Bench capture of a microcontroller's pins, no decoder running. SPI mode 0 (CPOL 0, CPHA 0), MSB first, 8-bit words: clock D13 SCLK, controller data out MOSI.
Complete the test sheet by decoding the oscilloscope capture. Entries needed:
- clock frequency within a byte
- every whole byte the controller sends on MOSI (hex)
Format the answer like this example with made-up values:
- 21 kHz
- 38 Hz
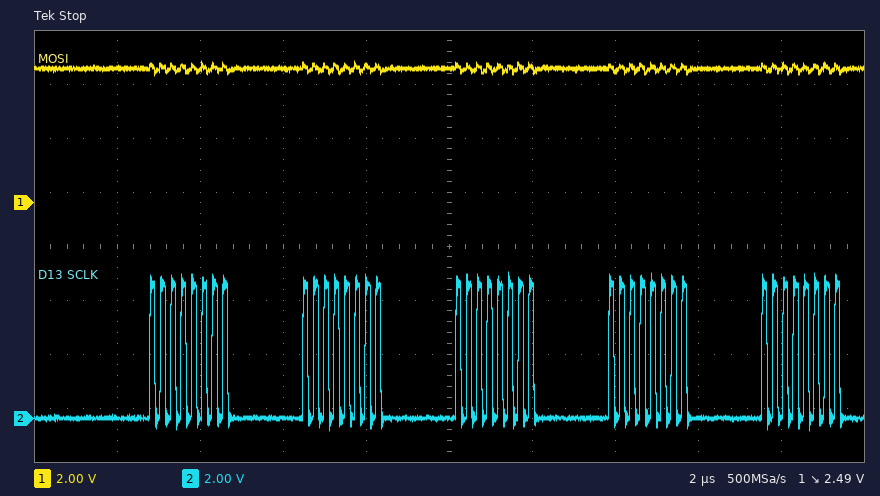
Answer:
- 4 MHz
- FF FF FF FF FF
